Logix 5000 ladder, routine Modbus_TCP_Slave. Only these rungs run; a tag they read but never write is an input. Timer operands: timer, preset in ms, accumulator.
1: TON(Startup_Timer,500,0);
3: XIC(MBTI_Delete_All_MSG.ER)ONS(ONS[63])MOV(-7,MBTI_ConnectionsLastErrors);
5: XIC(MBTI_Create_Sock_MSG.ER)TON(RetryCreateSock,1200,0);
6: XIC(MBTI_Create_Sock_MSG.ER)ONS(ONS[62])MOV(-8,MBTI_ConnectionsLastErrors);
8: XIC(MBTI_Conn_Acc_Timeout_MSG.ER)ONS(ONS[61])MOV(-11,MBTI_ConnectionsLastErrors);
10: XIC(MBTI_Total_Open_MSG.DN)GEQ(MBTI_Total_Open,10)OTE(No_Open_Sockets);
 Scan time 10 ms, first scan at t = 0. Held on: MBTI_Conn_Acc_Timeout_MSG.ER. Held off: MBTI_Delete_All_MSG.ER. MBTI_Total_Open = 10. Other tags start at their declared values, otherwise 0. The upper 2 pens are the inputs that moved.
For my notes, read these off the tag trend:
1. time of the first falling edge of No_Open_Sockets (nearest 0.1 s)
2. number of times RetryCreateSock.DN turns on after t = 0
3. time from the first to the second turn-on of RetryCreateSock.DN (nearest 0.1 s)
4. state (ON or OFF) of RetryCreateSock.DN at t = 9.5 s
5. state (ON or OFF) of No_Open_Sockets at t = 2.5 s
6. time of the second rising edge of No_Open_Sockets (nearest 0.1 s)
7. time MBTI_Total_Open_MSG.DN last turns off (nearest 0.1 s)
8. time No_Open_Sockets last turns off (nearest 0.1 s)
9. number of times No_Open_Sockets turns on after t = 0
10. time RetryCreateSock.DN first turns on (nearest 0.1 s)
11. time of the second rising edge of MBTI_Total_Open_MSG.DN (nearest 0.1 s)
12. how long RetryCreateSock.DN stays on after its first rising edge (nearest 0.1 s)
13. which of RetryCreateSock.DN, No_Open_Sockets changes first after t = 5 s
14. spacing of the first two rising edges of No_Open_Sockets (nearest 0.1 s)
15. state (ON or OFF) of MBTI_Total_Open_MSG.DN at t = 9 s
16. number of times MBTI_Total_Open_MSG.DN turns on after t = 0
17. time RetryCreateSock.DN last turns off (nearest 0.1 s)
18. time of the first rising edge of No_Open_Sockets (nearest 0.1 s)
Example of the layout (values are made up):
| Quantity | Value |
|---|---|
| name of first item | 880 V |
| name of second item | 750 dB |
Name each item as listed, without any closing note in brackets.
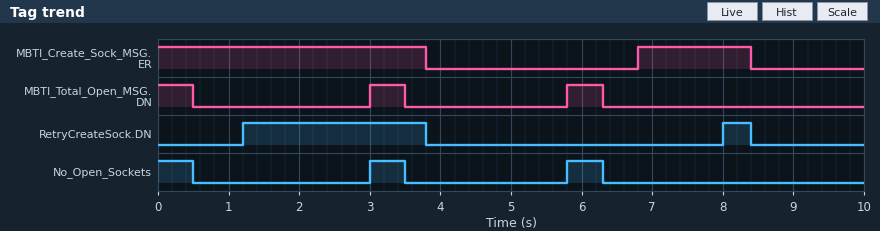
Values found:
| Quantity | Value |
|---|---|
| time of the first falling edge of No_Open_Sockets | 0.5 s |
| number of times RetryCreateSock.DN turns on after t = 0 | 2 |
| time from the first to the second turn-on of RetryCreateSock.DN | 6.8 s |
| state (ON or OFF) of RetryCreateSock.DN at t = 9.5 s | OFF |
| state (ON or OFF) of No_Open_Sockets at t = 2.5 s | OFF |
| time of the second rising edge of No_Open_Sockets | 5.8 s |
| time MBTI_Total_Open_MSG.DN last turns off | 6.3 s |
| time No_Open_Sockets last turns off | 6.3 s |
| number of times No_Open_Sockets turns on after t = 0 | 2 |
| time RetryCreateSock.DN first turns on | 1.2 s |
| time of the second rising edge of MBTI_Total_Open_MSG.DN | 5.8 s |
| how long RetryCreateSock.DN stays on after its first rising edge | 2.6 s |
| which of RetryCreateSock.DN, No_Open_Sockets changes first after t = 5 s | No_Open_Sockets |
| spacing of the first two rising edges of No_Open_Sockets | 2.8 s |
| state (ON or OFF) of MBTI_Total_Open_MSG.DN at t = 9 s | OFF |
| number of times MBTI_Total_Open_MSG.DN turns on after t = 0 | 2 |
| time RetryCreateSock.DN last turns off | 8.4 s |
| time of the first rising edge of No_Open_Sockets | 3.0 s |
